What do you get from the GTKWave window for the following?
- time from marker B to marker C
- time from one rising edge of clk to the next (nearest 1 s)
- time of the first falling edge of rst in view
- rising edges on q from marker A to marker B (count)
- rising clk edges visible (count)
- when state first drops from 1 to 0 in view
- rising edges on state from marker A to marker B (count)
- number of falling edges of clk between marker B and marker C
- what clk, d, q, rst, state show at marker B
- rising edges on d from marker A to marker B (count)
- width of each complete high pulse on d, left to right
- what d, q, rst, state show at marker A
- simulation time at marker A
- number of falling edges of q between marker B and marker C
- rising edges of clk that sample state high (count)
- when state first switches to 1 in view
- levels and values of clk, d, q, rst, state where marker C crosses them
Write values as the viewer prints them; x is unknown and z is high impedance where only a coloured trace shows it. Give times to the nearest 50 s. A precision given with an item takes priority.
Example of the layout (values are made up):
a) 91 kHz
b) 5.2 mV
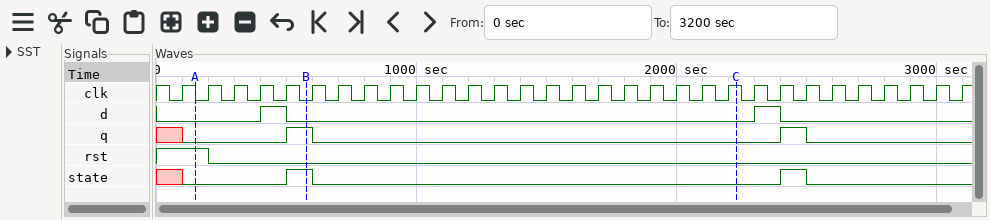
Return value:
a) 1650 s
b) 100 s
c) 200 s
d) 1
e) 31
f) 600 s
g) 1
h) 16
i) clk=0, d=0, q=1, rst=0, state=1
j) 1
k) 100 s, 100 s
l) d=0, q=0, rst=1, state=0
m) 150 s
n) 1
o) 2
p) 500 s
q) clk=1, d=0, q=0, rst=0, state=0
